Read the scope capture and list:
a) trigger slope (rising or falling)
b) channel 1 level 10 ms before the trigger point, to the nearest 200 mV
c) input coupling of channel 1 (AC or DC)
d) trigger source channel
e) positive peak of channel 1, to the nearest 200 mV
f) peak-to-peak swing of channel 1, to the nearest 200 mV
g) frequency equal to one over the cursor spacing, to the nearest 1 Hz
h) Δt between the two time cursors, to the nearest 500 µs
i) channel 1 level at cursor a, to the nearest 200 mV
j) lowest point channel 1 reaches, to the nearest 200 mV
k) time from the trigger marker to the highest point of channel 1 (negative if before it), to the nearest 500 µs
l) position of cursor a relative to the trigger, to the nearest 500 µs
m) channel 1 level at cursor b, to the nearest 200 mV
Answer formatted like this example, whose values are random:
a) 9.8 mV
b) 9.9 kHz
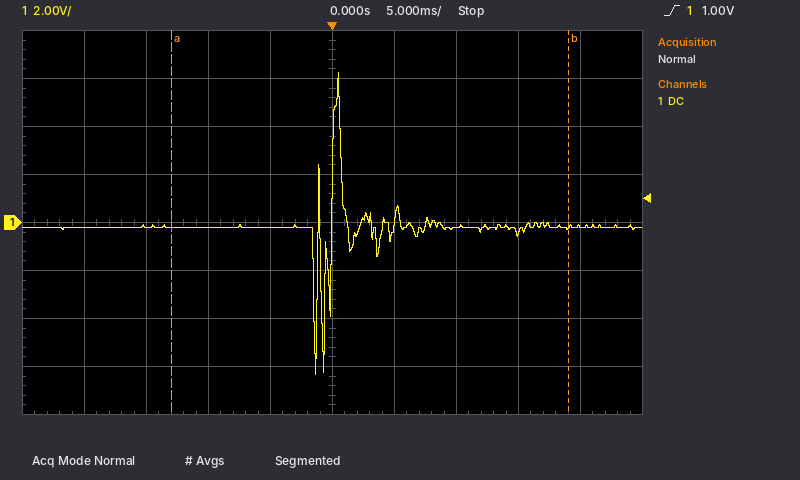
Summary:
a) rising
b) -200 mV
c) DC
d) channel 1
e) 6.2 V
f) 12.6 V
g) 31 Hz
h) 32.0 ms
i) -200 mV
j) -6.4 V
k) +500 µs
l) -13.0 ms
m) -200 mV
